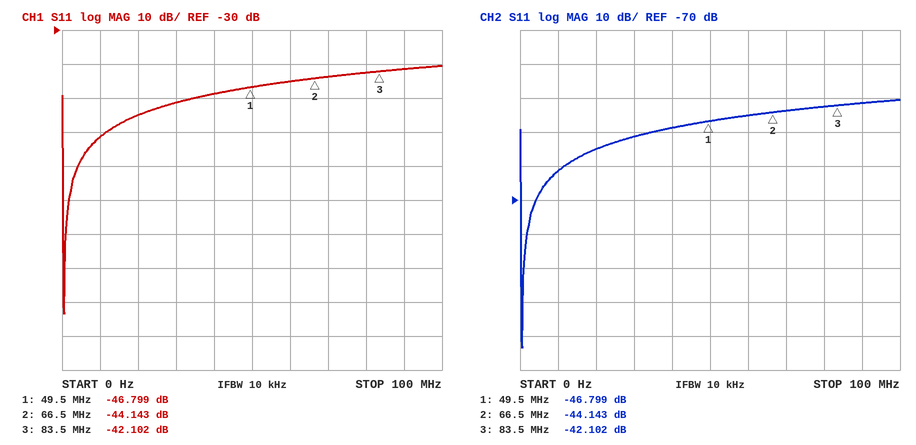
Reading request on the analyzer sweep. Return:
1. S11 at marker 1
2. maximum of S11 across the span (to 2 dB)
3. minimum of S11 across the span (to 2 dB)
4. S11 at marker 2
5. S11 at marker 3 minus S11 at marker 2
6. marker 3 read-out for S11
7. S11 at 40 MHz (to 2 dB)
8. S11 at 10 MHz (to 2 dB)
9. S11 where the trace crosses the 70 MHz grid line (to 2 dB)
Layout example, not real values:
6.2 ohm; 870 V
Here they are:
-46.799 dB; -40 dB; -114 dB; -44.143 dB; 2.041 dB; -42.102 dB; -48 dB; -62 dB; -44 dB
